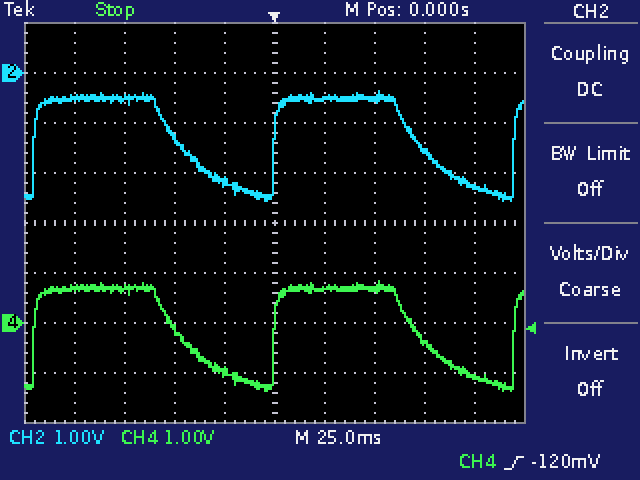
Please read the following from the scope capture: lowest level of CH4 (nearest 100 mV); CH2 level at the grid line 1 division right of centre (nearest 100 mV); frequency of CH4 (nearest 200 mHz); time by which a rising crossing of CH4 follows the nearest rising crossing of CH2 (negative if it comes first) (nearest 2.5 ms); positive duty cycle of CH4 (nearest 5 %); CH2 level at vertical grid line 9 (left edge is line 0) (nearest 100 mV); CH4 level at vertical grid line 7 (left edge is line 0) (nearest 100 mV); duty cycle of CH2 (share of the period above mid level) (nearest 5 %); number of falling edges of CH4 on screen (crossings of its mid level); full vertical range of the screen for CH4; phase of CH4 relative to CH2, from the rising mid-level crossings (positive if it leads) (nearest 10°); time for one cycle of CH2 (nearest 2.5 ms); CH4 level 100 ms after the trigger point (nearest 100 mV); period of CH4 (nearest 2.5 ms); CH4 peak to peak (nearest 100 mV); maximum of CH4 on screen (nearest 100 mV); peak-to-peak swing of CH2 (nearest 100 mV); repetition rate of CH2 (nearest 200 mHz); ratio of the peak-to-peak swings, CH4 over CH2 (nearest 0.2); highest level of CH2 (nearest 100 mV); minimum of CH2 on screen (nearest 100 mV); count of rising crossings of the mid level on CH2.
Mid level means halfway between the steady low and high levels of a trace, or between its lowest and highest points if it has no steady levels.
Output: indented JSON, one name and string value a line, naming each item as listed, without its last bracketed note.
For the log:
{
  "lowest level of CH4": "-1.4 V",
  "CH2 level at the grid line 1 division right of centre": "-500 mV",
  "frequency of CH4": "8.4 Hz",
  "time by which a rising crossing of CH4 follows the nearest rising crossing of CH2 (negative if it comes first)": "0.0 ms",
  "positive duty cycle of CH4": "60 %",
  "CH2 level at vertical grid line 9 (left edge is line 0)": "-2.3 V",
  "CH4 level at vertical grid line 7 (left edge is line 0)": "700 mV",
  "duty cycle of CH2 (share of the period above mid level)": "60 %",
  "number of falling edges of CH4 on screen": "2",
  "full vertical range of the screen for CH4": "8 V",
  "phase of CH4 relative to CH2, from the rising mid-level crossings (positive if it leads)": "0°",
  "time for one cycle of CH2": "120.0 ms",
  "CH4 level 100 ms after the trigger point": "-1.1 V",
  "period of CH4": "120.0 ms",
  "CH4 peak to peak": "2.2 V",
  "maximum of CH4 on screen": "800 mV",
  "peak-to-peak swing of CH2": "2.2 V",
  "repetition rate of CH2": "8.4 Hz",
  "ratio of the peak-to-peak swings, CH4 over CH2": "1.0",
  "highest level of CH2": "-400 mV",
  "minimum of CH2 on screen": "-2.6 V",
  "count of rising crossings of the mid level on CH2": "3"
}
